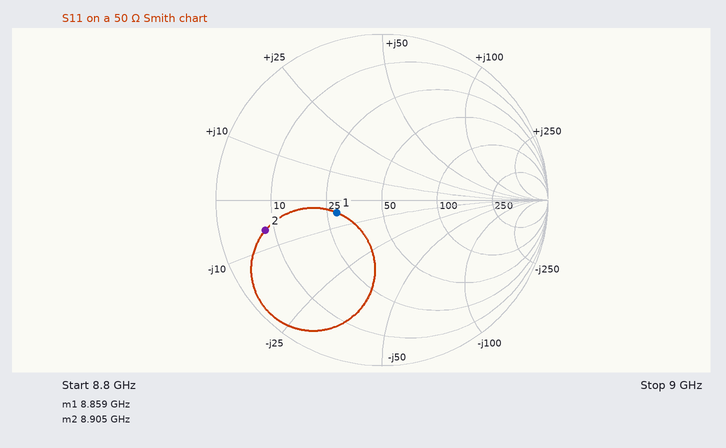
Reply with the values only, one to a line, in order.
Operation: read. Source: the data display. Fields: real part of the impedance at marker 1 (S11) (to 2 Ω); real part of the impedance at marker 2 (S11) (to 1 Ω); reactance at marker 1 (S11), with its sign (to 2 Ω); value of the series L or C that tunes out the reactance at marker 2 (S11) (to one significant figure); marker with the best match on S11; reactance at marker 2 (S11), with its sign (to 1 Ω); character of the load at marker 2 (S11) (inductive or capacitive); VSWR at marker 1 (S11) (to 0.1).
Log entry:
28 Ω
8 Ω
-4 Ω
100 pH
marker 1
-6 Ω
capacitive
1.8
